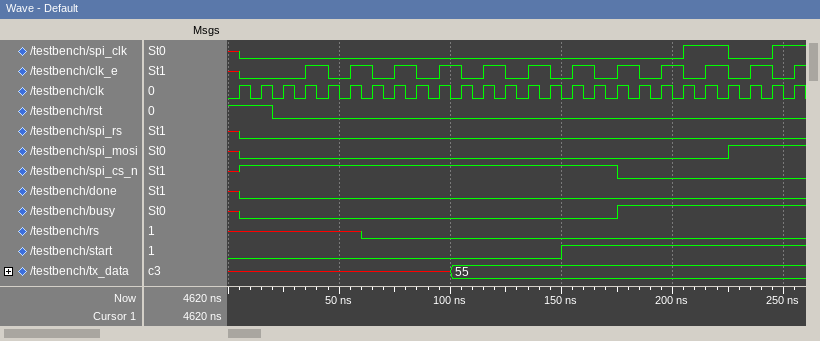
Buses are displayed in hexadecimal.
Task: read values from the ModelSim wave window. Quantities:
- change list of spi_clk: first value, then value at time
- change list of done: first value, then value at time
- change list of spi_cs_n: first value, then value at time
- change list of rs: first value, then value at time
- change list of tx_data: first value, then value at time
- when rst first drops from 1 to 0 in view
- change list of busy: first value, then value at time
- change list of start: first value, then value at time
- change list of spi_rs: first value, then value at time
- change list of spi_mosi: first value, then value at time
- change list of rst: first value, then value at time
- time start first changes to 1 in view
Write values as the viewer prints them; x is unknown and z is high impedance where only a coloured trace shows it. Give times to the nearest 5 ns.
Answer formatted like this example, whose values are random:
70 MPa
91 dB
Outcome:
x, 0 at 5 ns, 1 at 205 ns, 0 at 225 ns, 1 at 245 ns
x, 0 at 5 ns
x, 1 at 5 ns, 0 at 175 ns
x, 0 at 60 ns
x, 55 at 100 ns
20 ns
x, 0 at 5 ns, 1 at 175 ns
0, 1 at 150 ns
x, 0 at 5 ns
x, 0 at 5 ns, 1 at 225 ns
1, 0 at 20 ns
150 ns
